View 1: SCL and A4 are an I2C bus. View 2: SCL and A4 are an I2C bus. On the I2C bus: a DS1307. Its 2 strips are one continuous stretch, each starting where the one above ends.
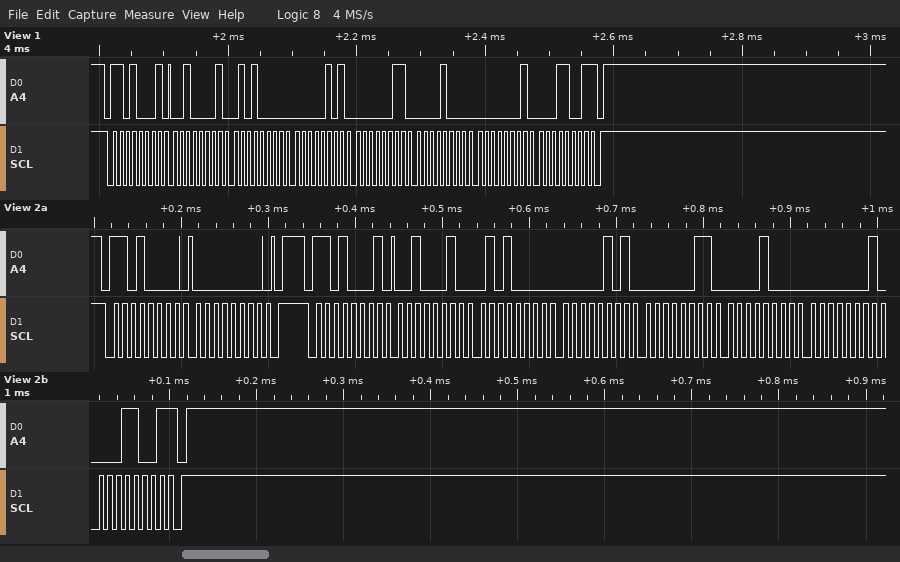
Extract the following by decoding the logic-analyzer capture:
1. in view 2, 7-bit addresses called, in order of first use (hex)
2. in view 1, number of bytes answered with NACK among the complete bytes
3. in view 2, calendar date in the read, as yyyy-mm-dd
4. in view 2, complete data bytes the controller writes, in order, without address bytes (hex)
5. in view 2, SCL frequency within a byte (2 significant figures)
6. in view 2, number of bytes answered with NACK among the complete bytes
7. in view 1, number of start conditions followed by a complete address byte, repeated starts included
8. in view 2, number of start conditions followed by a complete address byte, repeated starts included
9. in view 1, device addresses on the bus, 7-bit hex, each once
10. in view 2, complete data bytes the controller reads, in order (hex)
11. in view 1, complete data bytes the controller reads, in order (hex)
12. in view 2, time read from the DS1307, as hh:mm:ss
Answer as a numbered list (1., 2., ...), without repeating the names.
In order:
1. 0x68
2. 1
3. 2019-01-08
4. 00
5. 100 kHz
6. 1
7. 1
8. 2
9. 0x68
10. 22 50 05 03 08 01 19
11. 21 50 05 03 08 01 19
12. 05:50:22
